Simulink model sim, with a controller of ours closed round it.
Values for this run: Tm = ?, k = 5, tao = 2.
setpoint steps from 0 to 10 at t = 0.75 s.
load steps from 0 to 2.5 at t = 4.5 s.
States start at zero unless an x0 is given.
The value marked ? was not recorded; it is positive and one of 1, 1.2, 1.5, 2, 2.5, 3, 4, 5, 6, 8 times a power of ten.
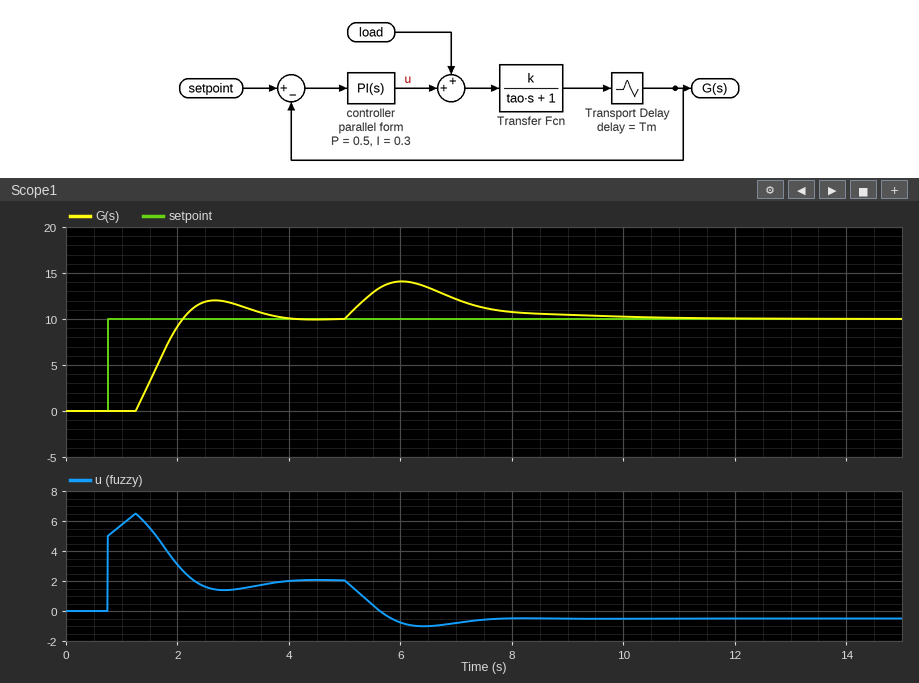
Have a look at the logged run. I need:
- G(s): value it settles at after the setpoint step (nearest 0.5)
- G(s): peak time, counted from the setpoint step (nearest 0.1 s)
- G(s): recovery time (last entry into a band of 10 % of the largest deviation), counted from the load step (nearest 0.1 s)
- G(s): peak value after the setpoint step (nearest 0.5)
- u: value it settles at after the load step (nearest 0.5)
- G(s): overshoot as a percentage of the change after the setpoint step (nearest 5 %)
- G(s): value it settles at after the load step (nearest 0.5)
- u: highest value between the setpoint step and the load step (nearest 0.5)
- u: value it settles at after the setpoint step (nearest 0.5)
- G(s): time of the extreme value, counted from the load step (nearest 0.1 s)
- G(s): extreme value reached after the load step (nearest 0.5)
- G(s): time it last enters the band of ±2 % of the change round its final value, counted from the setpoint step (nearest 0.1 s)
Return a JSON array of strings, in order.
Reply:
["10.0", "1.9 s", "4.7 s", "12.0", "-0.5", "20 %", "10.0", "6.5", "2.0", "1.5 s", "14.0", "3.1 s"]
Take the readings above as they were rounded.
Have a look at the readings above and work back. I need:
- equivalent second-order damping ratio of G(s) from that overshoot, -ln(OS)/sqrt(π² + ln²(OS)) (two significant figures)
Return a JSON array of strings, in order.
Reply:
["0.46"]
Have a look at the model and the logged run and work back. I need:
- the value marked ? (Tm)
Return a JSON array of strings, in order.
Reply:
["0.5"]
